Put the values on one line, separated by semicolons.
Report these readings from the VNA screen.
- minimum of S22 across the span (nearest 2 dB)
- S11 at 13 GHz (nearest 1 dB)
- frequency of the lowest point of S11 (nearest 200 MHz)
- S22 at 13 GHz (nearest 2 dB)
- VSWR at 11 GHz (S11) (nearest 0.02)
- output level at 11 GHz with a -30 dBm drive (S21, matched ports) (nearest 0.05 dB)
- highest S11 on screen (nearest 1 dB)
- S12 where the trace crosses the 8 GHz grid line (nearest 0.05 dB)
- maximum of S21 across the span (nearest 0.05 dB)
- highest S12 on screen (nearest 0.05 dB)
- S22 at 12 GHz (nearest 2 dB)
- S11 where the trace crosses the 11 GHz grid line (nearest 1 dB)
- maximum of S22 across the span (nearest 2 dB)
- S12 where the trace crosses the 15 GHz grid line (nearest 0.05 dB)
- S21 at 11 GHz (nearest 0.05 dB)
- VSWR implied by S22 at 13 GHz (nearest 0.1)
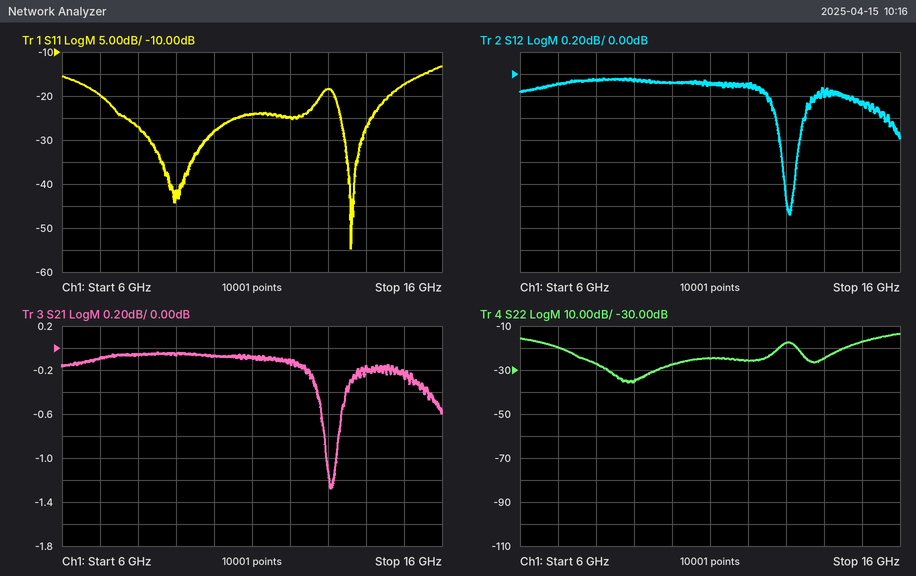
-36 dB; -18 dB; 13.6 GHz; -18 dB; 1.14; -30.10 dBm; -13 dB; -0.05 dB; -0.05 dB; -0.05 dB; -26 dB; -24 dB; -14 dB; -0.25 dB; -0.10 dB; 1.3
